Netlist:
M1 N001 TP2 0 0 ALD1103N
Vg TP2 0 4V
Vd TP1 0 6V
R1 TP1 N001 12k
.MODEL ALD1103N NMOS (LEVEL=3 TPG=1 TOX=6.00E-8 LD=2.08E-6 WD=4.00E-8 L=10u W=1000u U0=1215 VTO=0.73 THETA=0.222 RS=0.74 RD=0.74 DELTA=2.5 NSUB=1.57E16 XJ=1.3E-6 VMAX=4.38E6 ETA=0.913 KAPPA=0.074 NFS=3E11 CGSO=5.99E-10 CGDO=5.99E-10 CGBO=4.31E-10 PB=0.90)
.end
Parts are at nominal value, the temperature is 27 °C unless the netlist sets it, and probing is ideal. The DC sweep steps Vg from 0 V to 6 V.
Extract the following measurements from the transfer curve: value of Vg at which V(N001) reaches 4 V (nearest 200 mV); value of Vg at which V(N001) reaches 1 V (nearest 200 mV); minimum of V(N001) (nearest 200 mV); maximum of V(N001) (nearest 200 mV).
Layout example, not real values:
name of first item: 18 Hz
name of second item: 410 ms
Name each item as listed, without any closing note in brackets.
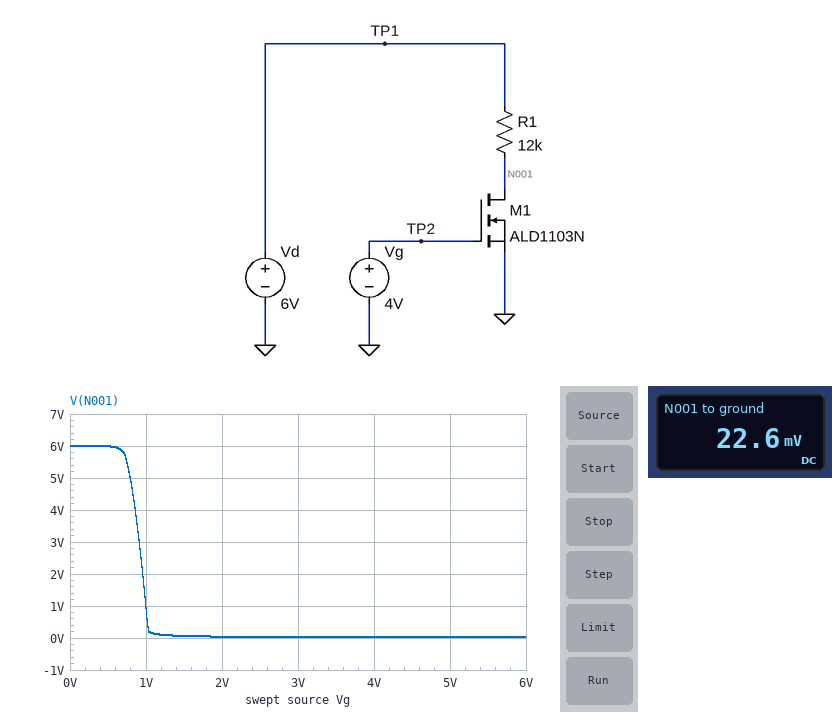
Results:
value of Vg at which V(N001) reaches 4 V: 800 mV
value of Vg at which V(N001) reaches 1 V: 1.0 V
minimum of V(N001): 0 V
maximum of V(N001): 6.0 V
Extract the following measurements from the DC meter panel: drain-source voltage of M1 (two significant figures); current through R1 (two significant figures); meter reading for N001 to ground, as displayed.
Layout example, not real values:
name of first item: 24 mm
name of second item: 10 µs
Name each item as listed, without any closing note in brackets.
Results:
drain-source voltage of M1: 23 mV
current through R1: 500 µA
meter reading for N001 to ground, as displayed: 22.6 mV
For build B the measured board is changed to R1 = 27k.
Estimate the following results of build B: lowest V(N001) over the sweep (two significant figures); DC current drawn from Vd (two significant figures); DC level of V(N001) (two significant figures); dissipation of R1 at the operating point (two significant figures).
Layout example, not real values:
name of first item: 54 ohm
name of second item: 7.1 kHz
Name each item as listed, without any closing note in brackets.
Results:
lowest V(N001) over the sweep: 7.9 mV
DC current drawn from Vd: 220 µA
DC level of V(N001): 10 mV
dissipation of R1 at the operating point: 1.3 mW
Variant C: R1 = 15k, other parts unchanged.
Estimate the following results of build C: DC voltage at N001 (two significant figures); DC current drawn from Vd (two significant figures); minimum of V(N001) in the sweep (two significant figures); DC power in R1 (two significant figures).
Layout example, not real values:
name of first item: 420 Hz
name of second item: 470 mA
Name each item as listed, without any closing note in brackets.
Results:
DC voltage at N001: 18 mV
DC current drawn from Vd: 400 µA
minimum of V(N001) in the sweep: 14 mV
DC power in R1: 2.4 mW
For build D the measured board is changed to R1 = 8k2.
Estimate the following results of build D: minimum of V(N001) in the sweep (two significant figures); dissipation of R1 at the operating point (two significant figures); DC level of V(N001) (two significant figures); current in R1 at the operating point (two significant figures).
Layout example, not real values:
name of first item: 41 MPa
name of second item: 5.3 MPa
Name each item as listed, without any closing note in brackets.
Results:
minimum of V(N001) in the sweep: 26 mV
dissipation of R1 at the operating point: 4.3 mW
DC level of V(N001): 33 mV
current in R1 at the operating point: 730 µA
